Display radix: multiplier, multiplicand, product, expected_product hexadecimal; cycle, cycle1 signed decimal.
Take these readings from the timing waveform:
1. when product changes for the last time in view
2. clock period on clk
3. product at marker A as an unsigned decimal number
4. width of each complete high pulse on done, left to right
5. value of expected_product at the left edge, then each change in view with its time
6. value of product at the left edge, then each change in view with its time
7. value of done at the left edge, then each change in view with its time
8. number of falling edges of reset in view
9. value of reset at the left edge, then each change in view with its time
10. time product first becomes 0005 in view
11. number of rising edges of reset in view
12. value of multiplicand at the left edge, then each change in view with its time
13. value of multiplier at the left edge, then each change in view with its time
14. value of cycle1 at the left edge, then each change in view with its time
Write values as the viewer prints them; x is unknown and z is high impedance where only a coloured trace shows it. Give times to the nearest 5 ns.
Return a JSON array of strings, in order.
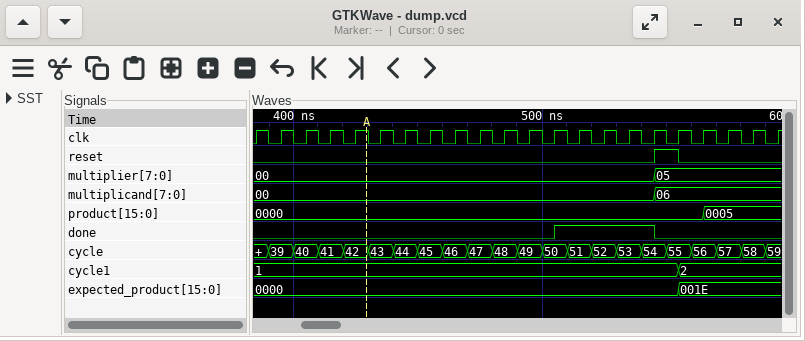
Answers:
["565 ns", "10 ns", "0", "40 ns", "0000, 001E at 555 ns", "0000, 0005 at 565 ns", "0, 1 at 505 ns, 0 at 545 ns", "1", "0, 1 at 545 ns, 0 at 555 ns", "565 ns", "1", "00, 06 at 545 ns", "00, 05 at 545 ns", "1, 2 at 555 ns"]
